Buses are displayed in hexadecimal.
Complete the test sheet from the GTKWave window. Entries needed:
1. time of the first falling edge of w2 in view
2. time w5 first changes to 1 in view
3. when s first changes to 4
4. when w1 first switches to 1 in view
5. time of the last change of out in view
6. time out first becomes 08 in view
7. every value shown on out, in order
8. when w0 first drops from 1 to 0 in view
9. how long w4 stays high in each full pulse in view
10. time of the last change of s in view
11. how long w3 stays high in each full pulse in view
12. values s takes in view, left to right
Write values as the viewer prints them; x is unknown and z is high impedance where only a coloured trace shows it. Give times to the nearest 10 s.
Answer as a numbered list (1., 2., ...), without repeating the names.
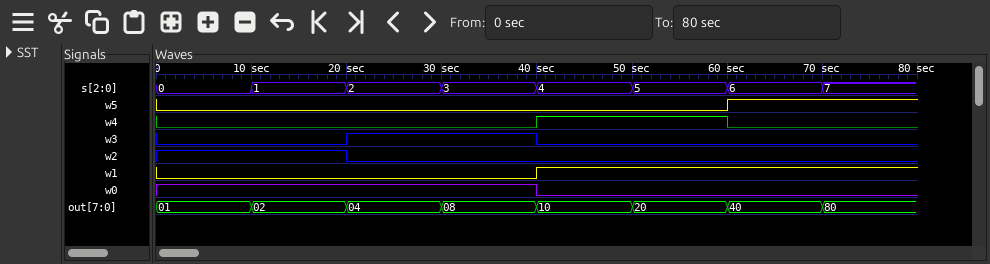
1. 20 s
2. 60 s
3. 40 s
4. 40 s
5. 70 s
6. 30 s
7. 01, 02, 04, 08, 10, 20, 40, 80
8. 40 s
9. 20 s
10. 70 s
11. 20 s
12. 0, 1, 2, 3, 4, 5, 6, 7
